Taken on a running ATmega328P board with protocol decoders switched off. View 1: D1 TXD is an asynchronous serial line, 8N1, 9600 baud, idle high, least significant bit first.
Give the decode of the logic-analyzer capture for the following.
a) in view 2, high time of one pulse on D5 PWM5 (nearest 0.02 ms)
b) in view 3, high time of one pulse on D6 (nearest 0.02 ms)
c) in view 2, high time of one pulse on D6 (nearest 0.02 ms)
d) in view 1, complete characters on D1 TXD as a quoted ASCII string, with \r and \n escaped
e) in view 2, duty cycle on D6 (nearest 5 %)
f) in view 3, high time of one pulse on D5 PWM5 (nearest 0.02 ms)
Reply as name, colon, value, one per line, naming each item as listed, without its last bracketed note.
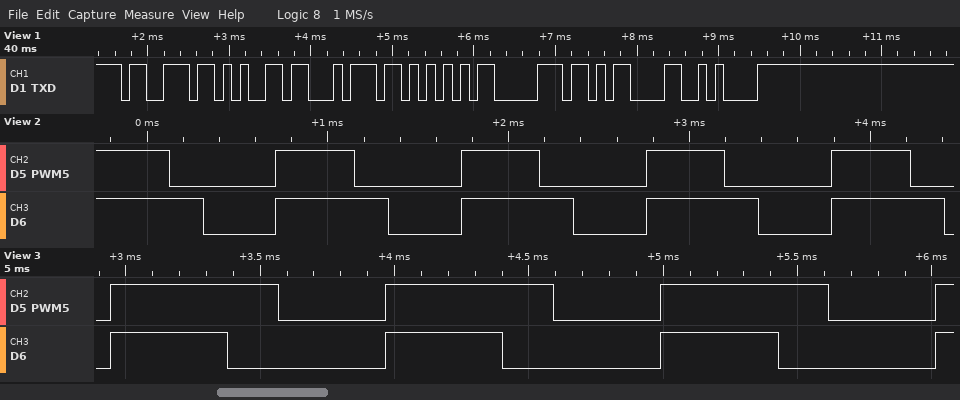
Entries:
in view 2, high time of one pulse on D5 PWM5: 0.44 ms
in view 3, high time of one pulse on D6: 0.44 ms
in view 2, high time of one pulse on D6: 0.62 ms
in view 1, complete characters on D1 TXD as a quoted ASCII string, with \r and \n escaped: "setUp\r\n"
in view 2, duty cycle on D6: 60 %
in view 3, high time of one pulse on D5 PWM5: 0.62 ms
